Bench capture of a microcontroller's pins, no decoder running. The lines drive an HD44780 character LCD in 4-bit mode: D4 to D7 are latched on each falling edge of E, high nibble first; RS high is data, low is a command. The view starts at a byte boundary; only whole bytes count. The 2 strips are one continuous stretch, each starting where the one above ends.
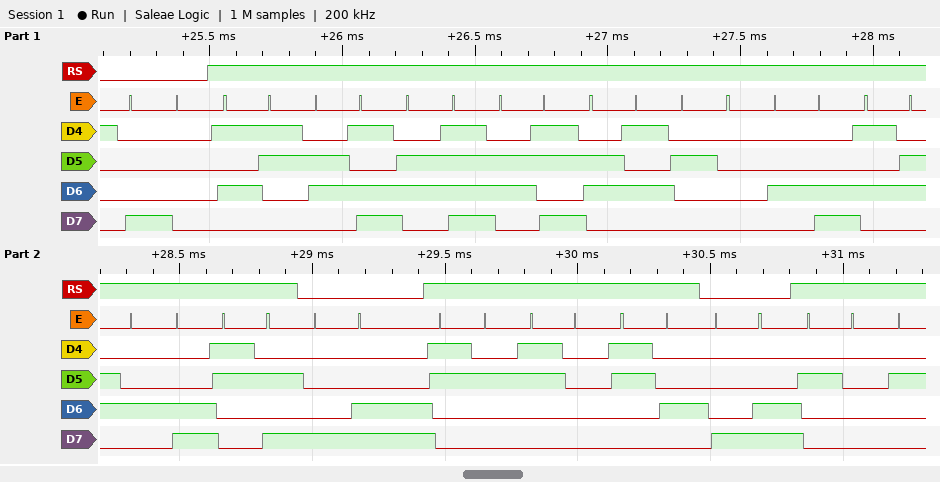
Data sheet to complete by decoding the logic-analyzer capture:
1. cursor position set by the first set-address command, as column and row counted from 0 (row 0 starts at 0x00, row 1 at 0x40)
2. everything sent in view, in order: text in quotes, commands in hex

column 0, row 0
0x80 "Smoke LVL:" 0x8C "204" 0x8C " "
